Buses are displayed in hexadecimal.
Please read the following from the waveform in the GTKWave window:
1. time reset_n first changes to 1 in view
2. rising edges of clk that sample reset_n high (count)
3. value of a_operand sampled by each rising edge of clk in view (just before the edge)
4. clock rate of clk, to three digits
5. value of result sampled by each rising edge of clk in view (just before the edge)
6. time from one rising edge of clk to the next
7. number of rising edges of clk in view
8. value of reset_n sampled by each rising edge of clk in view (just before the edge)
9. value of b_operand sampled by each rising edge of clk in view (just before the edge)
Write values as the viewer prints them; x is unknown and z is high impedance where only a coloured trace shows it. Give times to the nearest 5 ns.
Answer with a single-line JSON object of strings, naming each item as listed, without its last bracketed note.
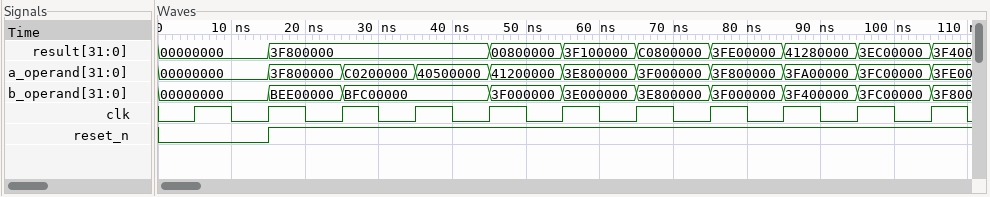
{"time reset_n first changes to 1 in view": "15 ns", "rising edges of clk that sample reset_n high": "9", "value of a_operand sampled by each rising edge of clk in view": "00000000, 00000000, 3F800000, C0200000, 40500000, 41200000, 3E800000, 3F000000, 3F800000, 3FA00000, 3FC00000", "clock rate of clk, to three digits": "100 MHz", "value of result sampled by each rising edge of clk in view": "00000000, 00000000, 3F800000, 3F800000, 3F800000, 00800000, 3F100000, C0800000, 3FE00000, 41280000, 3EC00000", "time from one rising edge of clk to the next": "10 ns", "number of rising edges of clk in view": "11", "value of reset_n sampled by each rising edge of clk in view": "0 0 1 1 1 1 1 1 1 1 1", "value of b_operand sampled by each rising edge of clk in view": "00000000, 00000000, BEE00000, BFC00000, BFC00000, 3F000000, 3E000000, 3E800000, 3F000000, 3F400000, 3FC00000"}
